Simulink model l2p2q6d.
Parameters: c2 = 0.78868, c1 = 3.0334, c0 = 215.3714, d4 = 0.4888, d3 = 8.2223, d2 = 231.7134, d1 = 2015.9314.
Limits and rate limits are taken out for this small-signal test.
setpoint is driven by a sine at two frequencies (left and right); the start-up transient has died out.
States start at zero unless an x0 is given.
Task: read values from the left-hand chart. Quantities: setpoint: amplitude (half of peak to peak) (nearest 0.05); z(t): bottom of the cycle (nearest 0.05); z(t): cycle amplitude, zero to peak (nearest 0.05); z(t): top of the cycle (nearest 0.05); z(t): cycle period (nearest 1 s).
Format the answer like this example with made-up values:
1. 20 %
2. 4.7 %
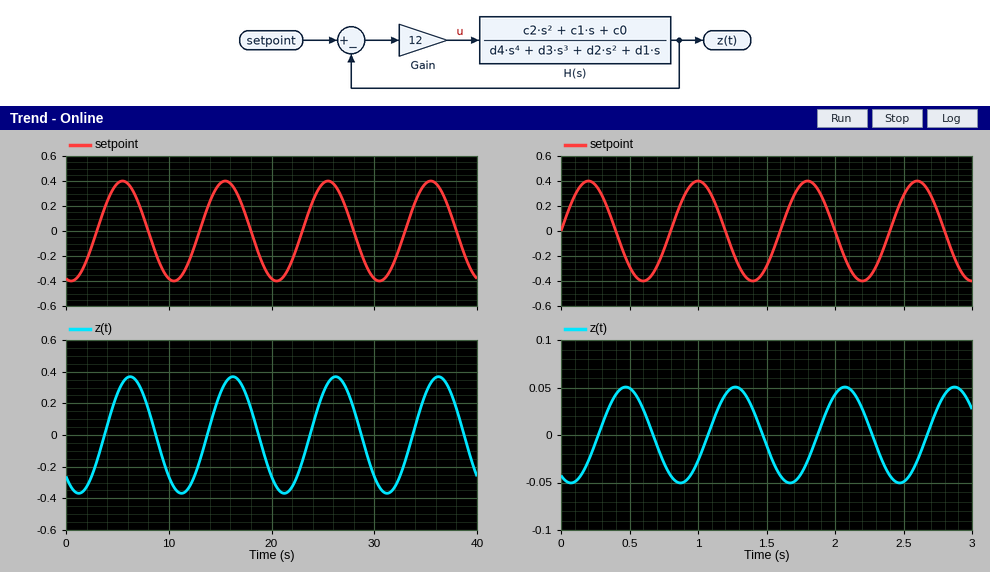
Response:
1. 0.40
2. -0.35
3. 0.35
4. 0.35
5. 10 s
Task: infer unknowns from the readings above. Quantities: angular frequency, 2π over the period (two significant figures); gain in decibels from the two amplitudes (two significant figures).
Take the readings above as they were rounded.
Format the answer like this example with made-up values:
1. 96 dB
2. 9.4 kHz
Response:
1. 0.63 rad/s
2. -1.2 dB
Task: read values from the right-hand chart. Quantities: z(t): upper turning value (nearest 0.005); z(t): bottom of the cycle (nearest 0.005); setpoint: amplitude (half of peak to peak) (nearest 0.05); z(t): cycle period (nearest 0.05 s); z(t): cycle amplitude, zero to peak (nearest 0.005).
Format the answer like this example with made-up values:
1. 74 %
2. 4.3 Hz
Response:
1. 0.050
2. -0.050
3. 0.40
4. 0.80 s
5. 0.050
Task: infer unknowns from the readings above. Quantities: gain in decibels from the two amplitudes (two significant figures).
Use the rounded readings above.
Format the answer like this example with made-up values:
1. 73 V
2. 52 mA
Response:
1. -18 dB
